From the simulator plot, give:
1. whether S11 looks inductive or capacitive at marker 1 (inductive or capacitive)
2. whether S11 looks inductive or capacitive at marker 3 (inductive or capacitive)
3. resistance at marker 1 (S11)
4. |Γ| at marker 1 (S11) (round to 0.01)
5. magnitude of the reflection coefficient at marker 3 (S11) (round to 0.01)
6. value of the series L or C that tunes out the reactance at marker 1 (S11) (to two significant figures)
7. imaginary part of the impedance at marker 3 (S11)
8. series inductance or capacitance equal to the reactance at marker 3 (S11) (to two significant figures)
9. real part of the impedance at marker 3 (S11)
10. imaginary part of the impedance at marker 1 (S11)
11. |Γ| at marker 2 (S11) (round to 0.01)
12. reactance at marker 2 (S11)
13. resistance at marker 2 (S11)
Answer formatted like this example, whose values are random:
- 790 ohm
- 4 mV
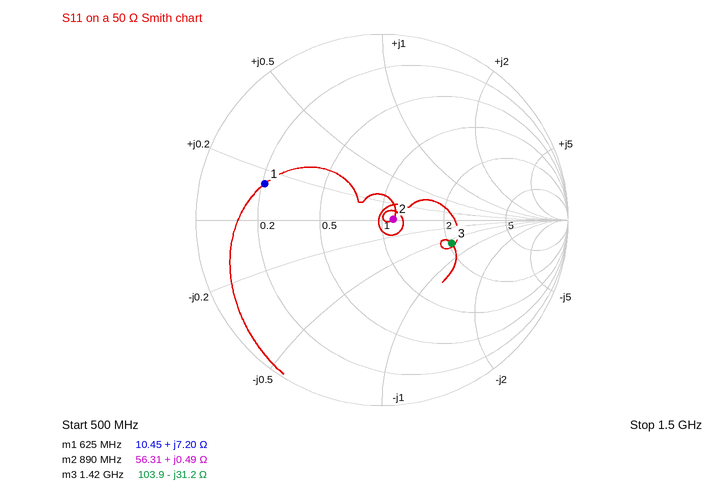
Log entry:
- inductive
- capacitive
- 10.45 Ω
- 0.66
- 0.40
- 35 pF
- -31.2 Ω
- 3.6 pF
- 103.9 Ω
- +7.20 Ω
- 0.06
- +0.49 Ω
- 56.31 Ω
